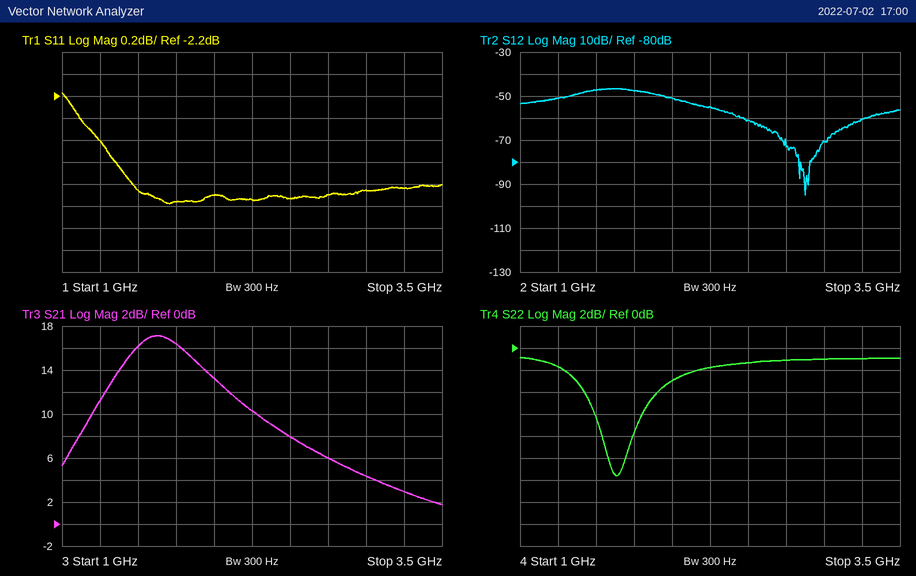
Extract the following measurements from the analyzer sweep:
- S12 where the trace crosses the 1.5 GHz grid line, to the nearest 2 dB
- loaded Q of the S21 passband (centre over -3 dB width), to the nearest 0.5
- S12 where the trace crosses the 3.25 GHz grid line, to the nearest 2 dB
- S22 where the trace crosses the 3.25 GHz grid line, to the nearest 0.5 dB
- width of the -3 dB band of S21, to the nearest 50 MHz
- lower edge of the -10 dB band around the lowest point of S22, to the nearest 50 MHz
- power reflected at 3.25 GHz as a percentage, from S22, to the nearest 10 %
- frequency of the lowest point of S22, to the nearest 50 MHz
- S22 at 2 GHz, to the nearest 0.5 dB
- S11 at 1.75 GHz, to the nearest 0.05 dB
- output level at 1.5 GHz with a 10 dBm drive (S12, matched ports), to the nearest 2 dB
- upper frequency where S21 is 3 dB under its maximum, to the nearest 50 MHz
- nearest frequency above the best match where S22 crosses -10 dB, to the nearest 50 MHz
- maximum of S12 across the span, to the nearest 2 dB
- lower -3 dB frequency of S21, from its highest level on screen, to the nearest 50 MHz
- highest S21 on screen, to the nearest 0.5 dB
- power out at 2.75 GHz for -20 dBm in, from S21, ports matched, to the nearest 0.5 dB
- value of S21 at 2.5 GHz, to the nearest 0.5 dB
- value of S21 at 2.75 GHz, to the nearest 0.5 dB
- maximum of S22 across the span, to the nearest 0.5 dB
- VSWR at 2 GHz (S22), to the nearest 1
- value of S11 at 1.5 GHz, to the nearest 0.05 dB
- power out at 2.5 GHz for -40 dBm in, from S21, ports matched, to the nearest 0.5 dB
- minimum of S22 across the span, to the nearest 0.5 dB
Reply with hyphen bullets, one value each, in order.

- -48 dB
- 3.0
- -60 dB
- -1.0 dB
- 550 MHz
- 1.60 GHz
- 80 %
- 1.65 GHz
- -3.0 dB
- -3.15 dB
- -38 dBm
- 1.95 GHz
- 1.70 GHz
- -46 dB
- 1.40 GHz
- 17.0 dB
- -14.0 dBm
- 8.0 dB
- 6.0 dB
- -1.0 dB
- 6
- -3.05 dB
- -32.0 dBm
- -11.5 dB
